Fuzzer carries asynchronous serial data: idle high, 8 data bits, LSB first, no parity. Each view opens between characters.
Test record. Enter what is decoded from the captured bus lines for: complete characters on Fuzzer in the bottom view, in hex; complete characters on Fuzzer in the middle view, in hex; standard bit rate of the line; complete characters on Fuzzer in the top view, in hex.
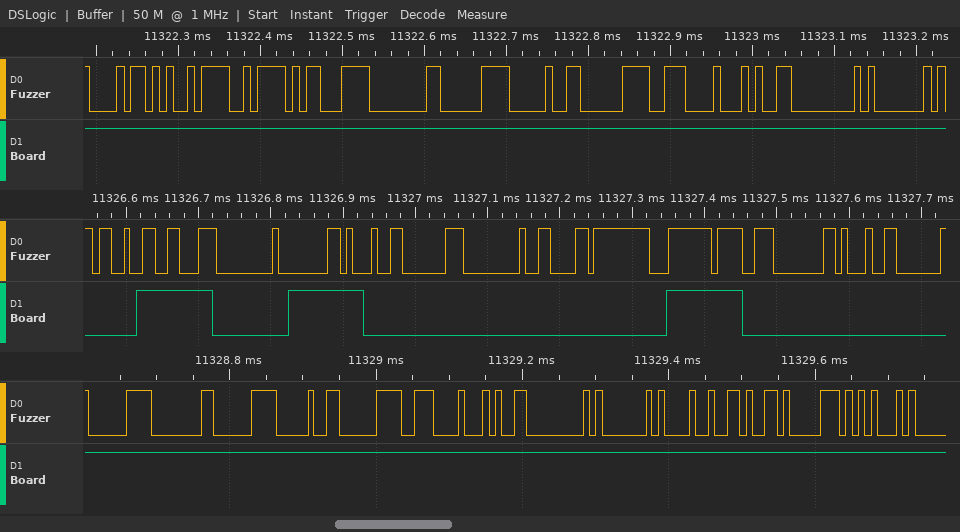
E0, 80, E0, 90, E0, 0E, 94, 00, 01, 21, 96, C1, 15
93, C6, 00, 80, 91, C0, 00, 86, FF, FC, CF, 80, 91
115200 baud
68, E9, 7A, E3, 80, E0, 90, E0, 0E, 94, 00, 01
